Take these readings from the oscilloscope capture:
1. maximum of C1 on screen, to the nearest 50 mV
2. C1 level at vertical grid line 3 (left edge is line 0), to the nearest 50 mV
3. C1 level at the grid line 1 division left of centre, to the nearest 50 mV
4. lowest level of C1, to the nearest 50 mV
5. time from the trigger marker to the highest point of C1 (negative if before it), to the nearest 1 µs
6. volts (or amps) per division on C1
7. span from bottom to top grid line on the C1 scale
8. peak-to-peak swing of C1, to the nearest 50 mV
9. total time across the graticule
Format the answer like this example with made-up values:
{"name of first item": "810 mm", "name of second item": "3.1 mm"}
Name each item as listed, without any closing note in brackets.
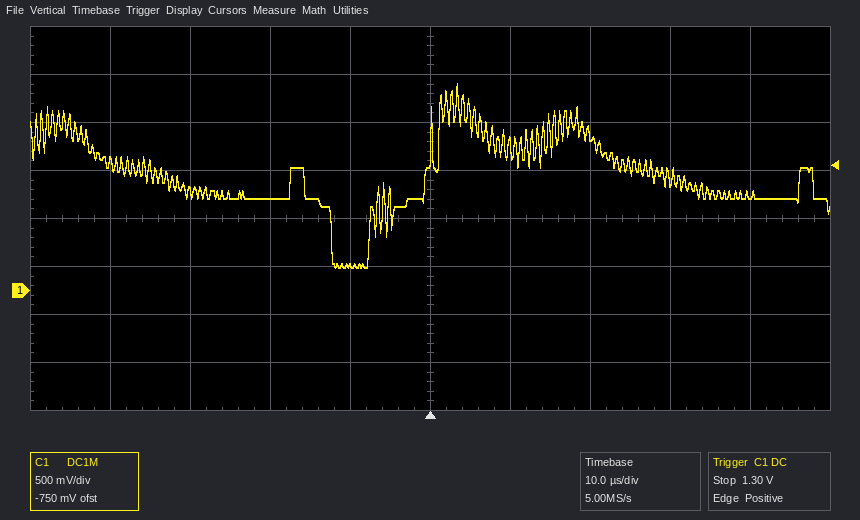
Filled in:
{"maximum of C1 on screen, to the nearest 50 mV": "2.15 V", "C1 level at vertical grid line 3 (left edge is line 0), to the nearest 50 mV": "950 mV", "C1 level at the grid line 1 division left of centre, to the nearest 50 mV": "250 mV", "lowest level of C1, to the nearest 50 mV": "250 mV", "time from the trigger marker to the highest point of C1 (negative if before it), to the nearest 1 µs": "+3 µs", "volts (or amps) per division on C1": "500 mV", "span from bottom to top grid line on the C1 scale": "4 V", "peak-to-peak swing of C1, to the nearest 50 mV": "1.90 V", "total time across the graticule": "100 µs"}
